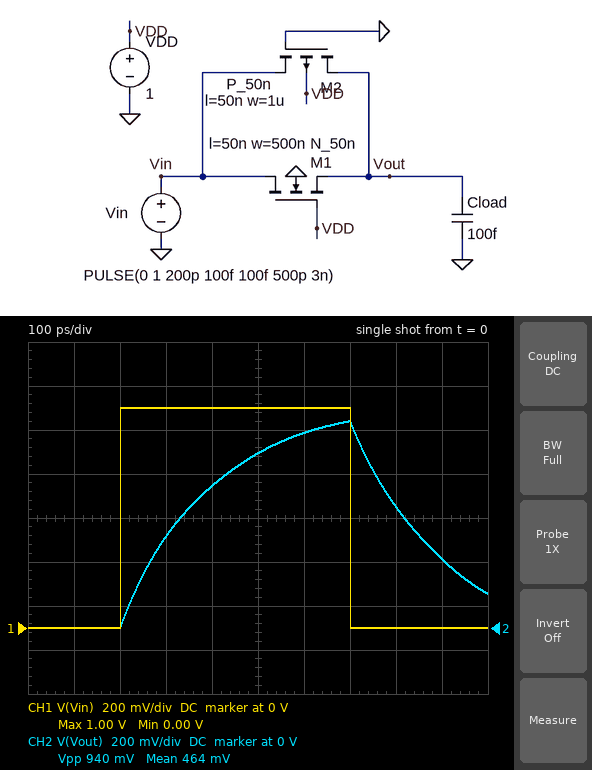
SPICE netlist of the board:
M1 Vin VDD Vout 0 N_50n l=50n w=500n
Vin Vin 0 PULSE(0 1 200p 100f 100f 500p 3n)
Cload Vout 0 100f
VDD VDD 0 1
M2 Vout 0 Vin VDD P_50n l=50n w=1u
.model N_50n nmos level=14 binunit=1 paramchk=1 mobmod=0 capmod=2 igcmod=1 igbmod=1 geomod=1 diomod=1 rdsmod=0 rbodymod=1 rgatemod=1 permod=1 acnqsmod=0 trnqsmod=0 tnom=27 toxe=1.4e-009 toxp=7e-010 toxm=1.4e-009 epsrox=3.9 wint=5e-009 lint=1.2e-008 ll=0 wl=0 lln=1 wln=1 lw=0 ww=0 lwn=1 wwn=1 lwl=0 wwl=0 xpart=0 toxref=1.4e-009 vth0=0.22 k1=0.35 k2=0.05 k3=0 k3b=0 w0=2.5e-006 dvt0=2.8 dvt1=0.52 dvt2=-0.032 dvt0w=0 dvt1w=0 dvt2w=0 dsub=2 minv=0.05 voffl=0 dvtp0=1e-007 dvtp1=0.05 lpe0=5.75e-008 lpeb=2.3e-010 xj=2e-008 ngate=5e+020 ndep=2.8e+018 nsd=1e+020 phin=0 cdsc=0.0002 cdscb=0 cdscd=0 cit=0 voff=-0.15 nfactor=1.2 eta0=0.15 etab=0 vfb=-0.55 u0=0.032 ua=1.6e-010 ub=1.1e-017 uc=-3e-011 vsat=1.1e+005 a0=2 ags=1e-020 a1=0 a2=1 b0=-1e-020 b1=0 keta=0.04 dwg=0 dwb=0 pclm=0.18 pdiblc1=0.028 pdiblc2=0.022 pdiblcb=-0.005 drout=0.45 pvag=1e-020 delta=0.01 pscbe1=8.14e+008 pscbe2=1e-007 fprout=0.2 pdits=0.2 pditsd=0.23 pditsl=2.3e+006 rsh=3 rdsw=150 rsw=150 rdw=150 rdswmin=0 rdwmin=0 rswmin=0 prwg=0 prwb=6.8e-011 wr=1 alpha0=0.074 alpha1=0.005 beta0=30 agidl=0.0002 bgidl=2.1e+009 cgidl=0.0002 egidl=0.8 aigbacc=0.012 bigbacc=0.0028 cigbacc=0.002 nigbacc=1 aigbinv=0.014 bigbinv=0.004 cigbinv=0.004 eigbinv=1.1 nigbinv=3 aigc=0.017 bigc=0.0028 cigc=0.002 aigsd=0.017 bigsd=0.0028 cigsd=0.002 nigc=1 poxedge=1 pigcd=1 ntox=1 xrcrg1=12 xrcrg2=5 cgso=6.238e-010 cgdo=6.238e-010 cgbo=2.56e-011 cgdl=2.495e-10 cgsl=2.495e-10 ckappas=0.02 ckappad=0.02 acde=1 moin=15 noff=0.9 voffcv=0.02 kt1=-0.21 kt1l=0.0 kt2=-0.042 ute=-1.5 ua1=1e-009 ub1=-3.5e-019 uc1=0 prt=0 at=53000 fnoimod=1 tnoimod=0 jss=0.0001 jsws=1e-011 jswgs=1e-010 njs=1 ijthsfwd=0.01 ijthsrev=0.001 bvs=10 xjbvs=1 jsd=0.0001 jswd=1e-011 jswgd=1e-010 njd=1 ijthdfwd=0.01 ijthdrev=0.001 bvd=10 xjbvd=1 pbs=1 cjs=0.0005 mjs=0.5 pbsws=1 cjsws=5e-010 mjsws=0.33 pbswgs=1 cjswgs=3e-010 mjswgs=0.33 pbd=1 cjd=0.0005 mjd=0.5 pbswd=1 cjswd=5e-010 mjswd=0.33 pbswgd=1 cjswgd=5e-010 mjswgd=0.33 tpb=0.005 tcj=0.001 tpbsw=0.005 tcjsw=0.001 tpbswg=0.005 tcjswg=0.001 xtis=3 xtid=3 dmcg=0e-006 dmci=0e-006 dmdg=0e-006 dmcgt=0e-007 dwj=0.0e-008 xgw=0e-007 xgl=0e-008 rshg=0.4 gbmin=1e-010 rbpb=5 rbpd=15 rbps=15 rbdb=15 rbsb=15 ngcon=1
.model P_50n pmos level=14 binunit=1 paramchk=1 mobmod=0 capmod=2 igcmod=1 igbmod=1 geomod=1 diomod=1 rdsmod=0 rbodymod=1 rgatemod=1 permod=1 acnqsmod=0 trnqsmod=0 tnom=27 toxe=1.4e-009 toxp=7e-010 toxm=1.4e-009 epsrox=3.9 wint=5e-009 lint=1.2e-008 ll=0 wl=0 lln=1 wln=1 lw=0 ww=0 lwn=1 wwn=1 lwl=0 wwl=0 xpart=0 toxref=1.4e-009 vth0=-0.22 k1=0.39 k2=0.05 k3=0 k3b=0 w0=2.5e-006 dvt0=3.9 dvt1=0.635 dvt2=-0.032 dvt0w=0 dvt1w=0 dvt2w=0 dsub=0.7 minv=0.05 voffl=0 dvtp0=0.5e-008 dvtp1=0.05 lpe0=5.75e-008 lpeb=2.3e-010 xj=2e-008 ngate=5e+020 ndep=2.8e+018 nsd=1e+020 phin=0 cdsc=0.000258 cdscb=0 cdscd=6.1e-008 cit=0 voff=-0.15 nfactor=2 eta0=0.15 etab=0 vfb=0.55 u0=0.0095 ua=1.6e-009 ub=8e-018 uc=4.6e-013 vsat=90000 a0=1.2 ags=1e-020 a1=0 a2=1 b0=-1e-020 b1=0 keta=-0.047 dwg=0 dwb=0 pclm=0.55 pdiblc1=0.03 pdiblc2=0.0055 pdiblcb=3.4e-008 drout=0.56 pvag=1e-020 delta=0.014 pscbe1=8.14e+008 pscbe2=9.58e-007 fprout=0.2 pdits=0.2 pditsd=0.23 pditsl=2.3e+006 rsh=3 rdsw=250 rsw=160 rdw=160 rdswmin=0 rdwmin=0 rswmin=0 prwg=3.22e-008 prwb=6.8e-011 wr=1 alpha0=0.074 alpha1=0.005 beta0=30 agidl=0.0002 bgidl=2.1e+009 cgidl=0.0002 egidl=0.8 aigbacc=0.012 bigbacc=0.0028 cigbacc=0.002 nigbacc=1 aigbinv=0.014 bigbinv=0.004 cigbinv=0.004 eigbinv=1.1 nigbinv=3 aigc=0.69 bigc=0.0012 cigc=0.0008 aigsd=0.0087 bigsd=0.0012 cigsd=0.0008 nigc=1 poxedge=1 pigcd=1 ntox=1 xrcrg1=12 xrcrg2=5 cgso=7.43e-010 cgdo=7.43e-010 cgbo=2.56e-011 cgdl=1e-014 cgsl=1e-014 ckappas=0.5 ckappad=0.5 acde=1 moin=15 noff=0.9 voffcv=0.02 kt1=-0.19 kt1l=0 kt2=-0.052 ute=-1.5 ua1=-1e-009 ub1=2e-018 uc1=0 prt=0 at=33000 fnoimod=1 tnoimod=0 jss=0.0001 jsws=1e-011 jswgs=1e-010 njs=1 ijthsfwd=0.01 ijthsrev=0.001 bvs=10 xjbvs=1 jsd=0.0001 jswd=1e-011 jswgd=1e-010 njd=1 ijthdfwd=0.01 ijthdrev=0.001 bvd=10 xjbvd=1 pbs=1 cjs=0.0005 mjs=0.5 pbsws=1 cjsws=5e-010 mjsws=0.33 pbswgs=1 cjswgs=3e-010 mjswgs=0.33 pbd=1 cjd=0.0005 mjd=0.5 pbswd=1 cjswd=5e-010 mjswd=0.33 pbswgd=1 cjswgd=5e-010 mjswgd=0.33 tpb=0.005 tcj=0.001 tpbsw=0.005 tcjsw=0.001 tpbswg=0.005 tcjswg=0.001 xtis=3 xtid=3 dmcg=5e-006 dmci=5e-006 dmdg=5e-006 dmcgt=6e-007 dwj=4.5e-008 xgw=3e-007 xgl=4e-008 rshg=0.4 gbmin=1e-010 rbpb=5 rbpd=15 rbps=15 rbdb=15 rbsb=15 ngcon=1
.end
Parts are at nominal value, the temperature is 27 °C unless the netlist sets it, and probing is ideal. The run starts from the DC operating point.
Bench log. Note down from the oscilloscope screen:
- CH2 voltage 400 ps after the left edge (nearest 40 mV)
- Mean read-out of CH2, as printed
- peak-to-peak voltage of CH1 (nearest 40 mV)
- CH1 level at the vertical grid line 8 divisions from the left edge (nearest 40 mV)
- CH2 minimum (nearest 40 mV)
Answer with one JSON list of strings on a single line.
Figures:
["640 mV", "464 mV", "1.00 V", "0 V", "0 V"]
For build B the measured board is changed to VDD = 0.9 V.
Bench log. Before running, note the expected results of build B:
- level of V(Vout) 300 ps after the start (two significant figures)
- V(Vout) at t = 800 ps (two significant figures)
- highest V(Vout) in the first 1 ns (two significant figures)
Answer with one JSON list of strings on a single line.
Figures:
["390 mV", "570 mV", "940 mV"]
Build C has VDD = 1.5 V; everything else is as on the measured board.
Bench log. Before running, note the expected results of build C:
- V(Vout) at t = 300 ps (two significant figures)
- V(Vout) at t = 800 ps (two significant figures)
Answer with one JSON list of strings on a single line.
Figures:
["530 mV", "490 mV"]
